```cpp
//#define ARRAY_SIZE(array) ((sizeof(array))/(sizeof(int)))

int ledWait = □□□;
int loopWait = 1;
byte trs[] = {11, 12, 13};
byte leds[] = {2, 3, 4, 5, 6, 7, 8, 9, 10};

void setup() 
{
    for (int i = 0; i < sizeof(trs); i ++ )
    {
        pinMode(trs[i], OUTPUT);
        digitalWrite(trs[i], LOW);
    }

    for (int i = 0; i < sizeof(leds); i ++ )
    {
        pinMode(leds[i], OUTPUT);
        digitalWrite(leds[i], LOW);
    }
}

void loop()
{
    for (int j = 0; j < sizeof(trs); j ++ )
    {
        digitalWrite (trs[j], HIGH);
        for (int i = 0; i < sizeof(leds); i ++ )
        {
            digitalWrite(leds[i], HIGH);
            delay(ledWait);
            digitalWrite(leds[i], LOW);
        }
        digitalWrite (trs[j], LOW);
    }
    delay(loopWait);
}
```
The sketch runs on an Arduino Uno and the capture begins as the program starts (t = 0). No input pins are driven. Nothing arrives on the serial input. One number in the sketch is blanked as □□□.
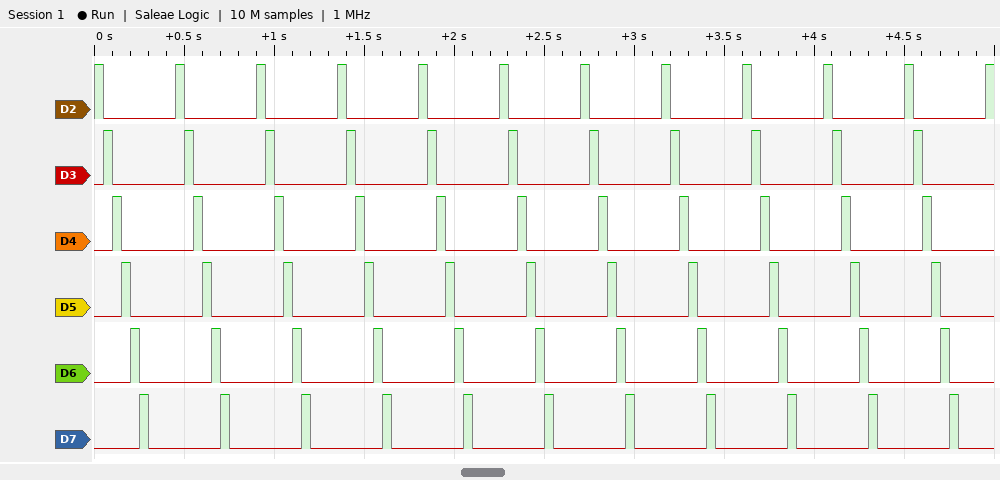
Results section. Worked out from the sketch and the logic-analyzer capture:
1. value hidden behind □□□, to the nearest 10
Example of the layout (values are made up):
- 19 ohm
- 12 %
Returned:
- 50
